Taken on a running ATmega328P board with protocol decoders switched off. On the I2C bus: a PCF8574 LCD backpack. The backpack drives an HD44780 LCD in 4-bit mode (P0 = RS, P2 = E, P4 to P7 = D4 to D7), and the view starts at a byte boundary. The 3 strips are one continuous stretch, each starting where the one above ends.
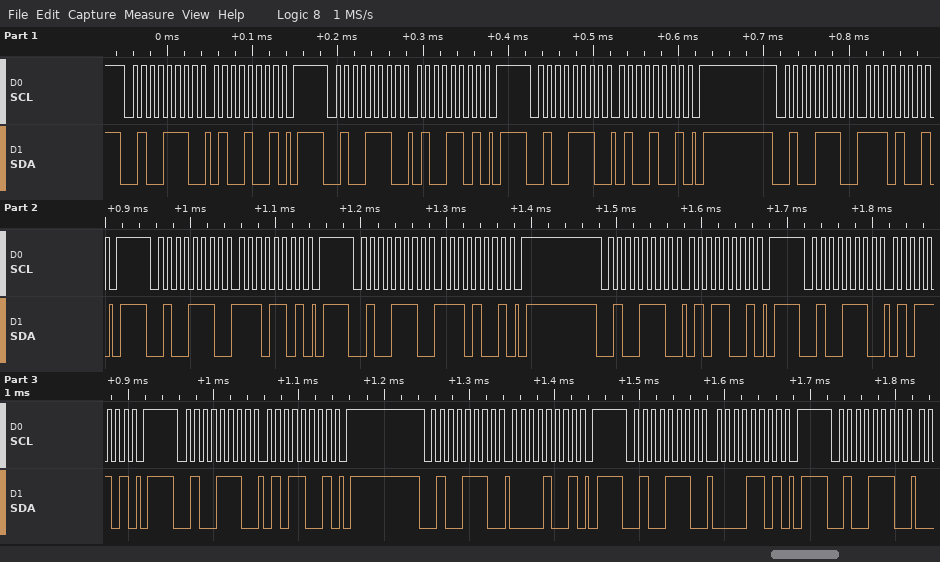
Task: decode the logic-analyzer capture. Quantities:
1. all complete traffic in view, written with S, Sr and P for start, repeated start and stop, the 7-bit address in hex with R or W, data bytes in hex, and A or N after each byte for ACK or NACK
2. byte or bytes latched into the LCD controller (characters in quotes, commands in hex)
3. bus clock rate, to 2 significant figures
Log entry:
S 27W A 49 A P S 27W A 4D A P S 27W A 49 A P S 27W A E9 A P S 27W A ED A P S 27W A E9 A P S 27W A 59 A P S 27W A 5D A P S 27W A 59 A P S 27W A 09 A P S 27W A 0D A P S 27W A
'N'
100 kHz
